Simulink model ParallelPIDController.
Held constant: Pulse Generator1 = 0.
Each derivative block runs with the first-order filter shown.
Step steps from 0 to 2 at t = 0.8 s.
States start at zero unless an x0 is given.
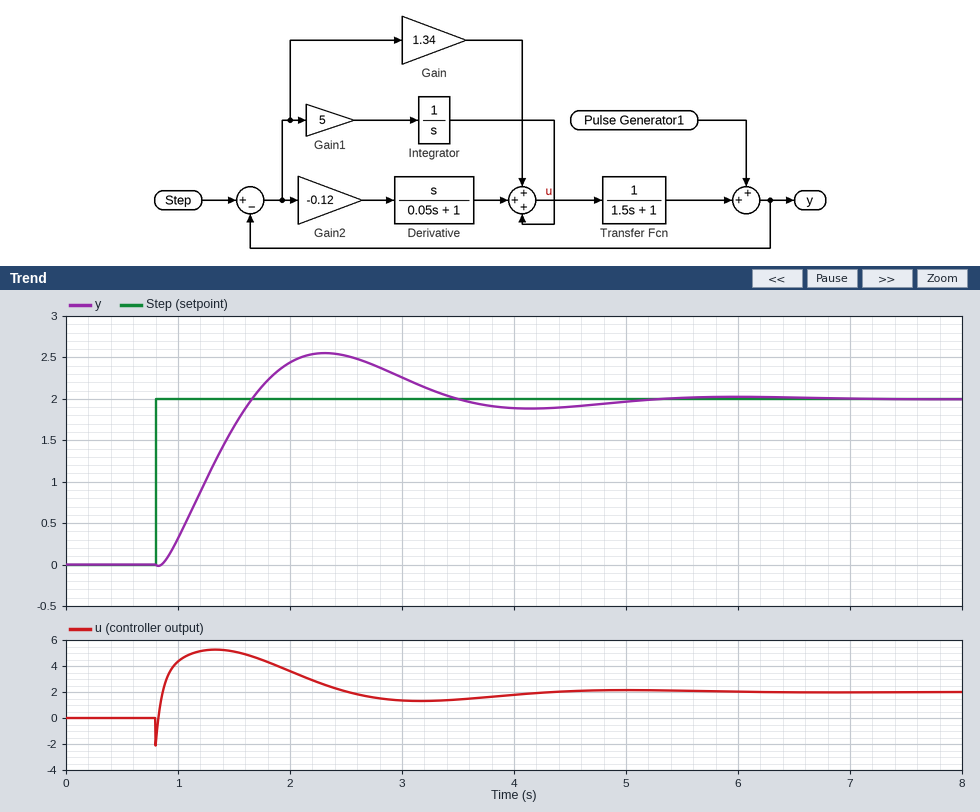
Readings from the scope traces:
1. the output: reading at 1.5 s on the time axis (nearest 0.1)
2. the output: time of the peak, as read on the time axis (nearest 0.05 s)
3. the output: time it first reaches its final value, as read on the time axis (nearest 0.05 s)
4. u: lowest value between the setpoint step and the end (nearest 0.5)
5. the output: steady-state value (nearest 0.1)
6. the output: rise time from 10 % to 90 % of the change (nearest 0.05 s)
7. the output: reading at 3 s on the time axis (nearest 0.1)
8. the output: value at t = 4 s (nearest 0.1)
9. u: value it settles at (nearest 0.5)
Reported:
1.7
2.30 s
1.65 s
-2.0
2.0
0.60 s
2.3
1.9
2.0
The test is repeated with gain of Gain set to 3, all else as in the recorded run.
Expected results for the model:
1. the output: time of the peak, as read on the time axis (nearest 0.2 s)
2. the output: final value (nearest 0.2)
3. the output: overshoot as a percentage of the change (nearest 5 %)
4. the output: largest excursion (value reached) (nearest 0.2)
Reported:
2.2 s
2.0
10 %
2.2
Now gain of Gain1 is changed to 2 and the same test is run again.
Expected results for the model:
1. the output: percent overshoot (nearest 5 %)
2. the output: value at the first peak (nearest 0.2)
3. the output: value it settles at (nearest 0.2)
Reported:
10 %
2.2
2.0
